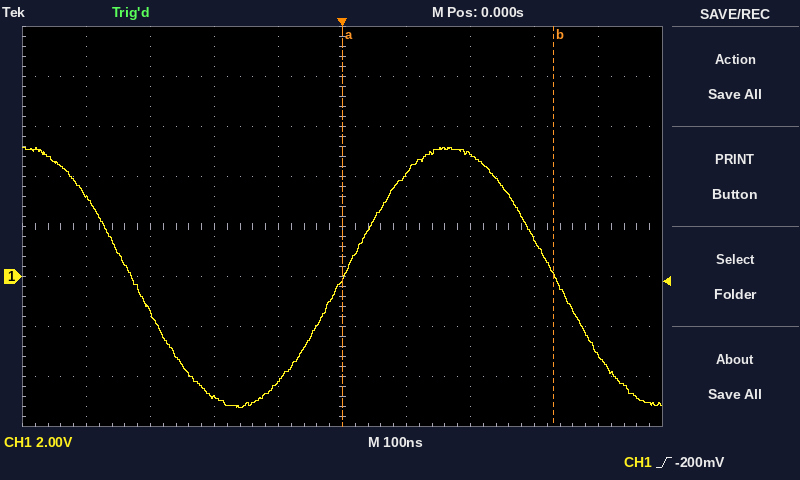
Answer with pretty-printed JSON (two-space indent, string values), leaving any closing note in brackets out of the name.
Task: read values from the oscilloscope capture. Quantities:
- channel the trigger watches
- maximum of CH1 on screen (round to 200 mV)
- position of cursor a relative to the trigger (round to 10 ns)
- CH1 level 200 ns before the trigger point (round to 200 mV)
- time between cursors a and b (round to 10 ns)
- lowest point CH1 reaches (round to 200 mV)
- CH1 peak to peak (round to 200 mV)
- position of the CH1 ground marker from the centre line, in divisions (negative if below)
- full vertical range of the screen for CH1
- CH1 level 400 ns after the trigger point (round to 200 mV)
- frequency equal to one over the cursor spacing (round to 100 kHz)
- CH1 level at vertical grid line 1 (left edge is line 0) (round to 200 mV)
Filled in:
{
  "channel the trigger watches": "CH1",
  "maximum of CH1 on screen": "5.2 V",
  "position of cursor a relative to the trigger": "0 ns",
  "CH1 level 200 ns before the trigger point": "-4.8 V",
  "time between cursors a and b": "330 ns",
  "lowest point CH1 reaches": "-5.2 V",
  "CH1 peak to peak": "10.4 V",
  "position of the CH1 ground marker from the centre line, in divisions": "-1.0 div",
  "full vertical range of the screen for CH1": "16 V",
  "CH1 level 400 ns after the trigger point": "-3.2 V",
  "frequency equal to one over the cursor spacing": "3.0 MHz",
  "CH1 level at vertical grid line 1 (left edge is line 0)": "3.2 V"
}
